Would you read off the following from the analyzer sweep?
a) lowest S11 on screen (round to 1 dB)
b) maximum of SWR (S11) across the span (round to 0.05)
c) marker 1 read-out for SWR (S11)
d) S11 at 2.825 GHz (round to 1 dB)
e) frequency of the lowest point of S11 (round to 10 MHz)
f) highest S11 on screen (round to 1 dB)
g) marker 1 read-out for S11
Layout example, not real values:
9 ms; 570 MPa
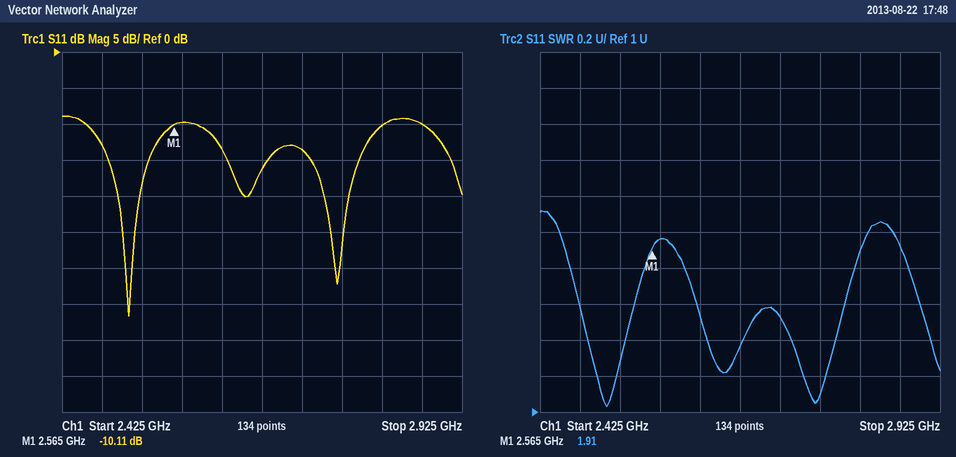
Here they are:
-37 dB; 2.10; 1.91; -10 dB; 2.51 GHz; -9 dB; -10.11 dB
